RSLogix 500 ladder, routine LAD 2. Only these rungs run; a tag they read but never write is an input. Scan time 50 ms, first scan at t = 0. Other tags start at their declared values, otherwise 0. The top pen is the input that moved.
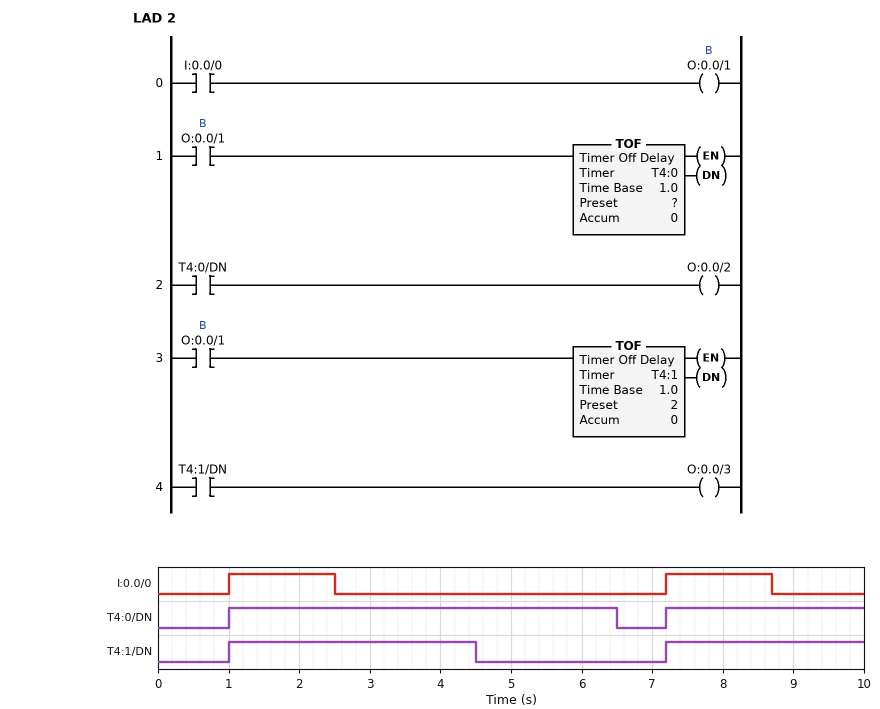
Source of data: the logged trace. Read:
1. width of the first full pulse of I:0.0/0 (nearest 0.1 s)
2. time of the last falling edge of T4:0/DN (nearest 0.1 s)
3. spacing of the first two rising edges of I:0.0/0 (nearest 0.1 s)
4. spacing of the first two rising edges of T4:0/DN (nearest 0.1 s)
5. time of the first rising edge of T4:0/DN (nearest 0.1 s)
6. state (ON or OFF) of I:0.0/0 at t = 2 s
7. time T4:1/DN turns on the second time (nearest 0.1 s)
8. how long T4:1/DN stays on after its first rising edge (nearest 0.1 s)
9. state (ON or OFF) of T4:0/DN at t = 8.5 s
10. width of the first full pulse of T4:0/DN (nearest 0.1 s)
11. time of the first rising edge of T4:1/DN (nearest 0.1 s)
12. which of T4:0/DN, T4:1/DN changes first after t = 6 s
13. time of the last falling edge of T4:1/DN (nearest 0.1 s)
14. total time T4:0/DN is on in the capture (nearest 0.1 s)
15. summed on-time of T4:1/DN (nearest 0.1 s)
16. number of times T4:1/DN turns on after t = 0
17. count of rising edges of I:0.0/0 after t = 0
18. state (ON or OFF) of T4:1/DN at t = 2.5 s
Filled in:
1.5 s
6.5 s
6.2 s
6.2 s
1.0 s
ON
7.2 s
3.5 s
ON
5.5 s
1.0 s
T4:0/DN
4.5 s
8.3 s
6.3 s
2
2
ON
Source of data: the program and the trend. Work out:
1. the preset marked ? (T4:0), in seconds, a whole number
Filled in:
4 s
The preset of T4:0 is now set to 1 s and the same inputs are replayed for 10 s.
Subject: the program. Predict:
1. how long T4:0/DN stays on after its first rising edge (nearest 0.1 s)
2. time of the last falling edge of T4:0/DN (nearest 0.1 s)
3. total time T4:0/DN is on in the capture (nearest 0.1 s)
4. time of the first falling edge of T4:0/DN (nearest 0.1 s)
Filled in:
2.5 s
9.7 s
5.0 s
3.5 s
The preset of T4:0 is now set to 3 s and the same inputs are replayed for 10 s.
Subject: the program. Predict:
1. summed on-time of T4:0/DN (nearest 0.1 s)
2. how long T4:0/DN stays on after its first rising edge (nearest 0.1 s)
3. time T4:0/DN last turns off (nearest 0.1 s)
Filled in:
7.3 s
4.5 s
5.5 s
